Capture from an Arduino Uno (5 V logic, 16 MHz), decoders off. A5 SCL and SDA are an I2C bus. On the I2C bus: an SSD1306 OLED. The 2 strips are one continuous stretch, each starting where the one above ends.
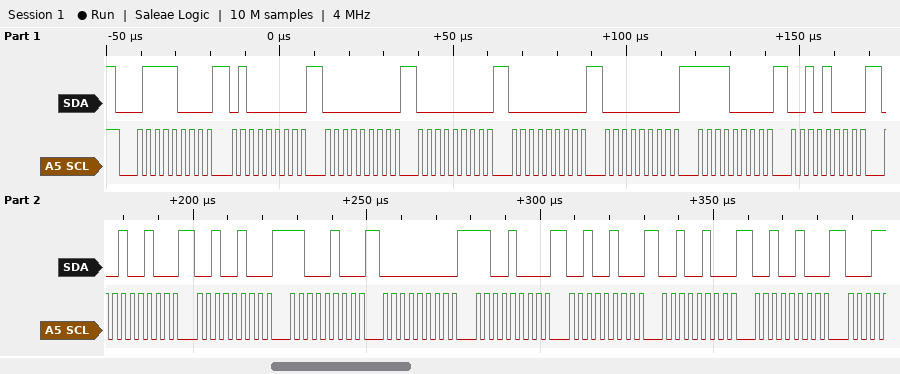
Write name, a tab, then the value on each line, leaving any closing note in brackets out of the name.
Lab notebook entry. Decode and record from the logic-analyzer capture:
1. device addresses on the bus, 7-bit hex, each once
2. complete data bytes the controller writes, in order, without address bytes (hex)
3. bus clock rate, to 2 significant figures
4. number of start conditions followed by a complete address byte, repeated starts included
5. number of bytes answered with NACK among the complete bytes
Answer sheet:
device addresses on the bus, 7-bit hex, each once	0x3C
complete data bytes the controller writes, in order, without address bytes	40 00 00 00 00 F0 28 24 24 C4 00 C8 24 24 24
bus clock rate, to 2 significant figures	400 kHz
number of start conditions followed by a complete address byte, repeated starts included	1
number of bytes answered with NACK among the complete bytes	0
